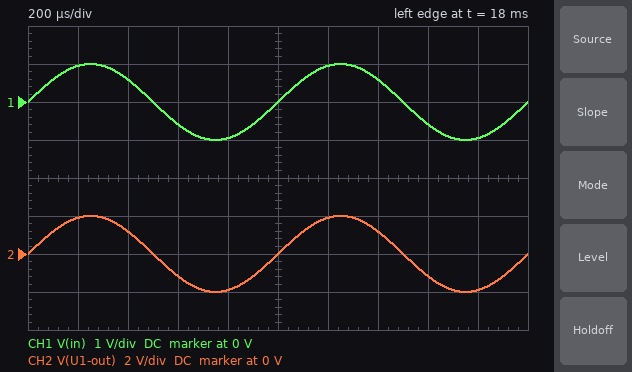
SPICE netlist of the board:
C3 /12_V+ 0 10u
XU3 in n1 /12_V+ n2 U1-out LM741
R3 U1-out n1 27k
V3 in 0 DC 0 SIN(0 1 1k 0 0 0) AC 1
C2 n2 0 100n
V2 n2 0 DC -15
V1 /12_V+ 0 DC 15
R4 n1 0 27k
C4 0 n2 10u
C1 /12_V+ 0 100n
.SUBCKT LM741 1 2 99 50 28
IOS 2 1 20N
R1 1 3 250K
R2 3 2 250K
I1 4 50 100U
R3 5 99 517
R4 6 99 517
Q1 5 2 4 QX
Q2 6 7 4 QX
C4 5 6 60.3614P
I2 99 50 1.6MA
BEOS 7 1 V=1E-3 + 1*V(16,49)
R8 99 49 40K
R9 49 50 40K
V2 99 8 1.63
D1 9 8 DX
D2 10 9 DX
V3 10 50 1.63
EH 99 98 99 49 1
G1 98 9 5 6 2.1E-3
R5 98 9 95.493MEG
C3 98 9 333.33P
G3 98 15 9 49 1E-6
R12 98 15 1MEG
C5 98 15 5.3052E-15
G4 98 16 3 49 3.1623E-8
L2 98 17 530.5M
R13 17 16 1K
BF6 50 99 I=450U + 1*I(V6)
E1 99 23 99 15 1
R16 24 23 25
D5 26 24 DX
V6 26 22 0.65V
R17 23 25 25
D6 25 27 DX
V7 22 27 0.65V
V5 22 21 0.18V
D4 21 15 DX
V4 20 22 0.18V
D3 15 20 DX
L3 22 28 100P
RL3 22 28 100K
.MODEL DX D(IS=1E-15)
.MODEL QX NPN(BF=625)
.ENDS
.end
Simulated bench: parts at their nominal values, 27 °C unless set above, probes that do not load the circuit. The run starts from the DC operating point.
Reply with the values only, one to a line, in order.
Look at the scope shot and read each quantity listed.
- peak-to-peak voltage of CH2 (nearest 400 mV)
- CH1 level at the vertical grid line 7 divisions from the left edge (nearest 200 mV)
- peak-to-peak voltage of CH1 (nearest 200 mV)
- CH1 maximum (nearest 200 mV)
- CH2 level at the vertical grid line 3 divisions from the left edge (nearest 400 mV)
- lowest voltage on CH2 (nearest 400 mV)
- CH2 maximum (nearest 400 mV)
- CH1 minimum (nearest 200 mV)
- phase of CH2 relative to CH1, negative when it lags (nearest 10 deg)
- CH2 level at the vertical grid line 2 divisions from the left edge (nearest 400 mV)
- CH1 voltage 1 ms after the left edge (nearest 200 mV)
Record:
4.0 V
600 mV
2.0 V
1.0 V
-1.2 V
-2.0 V
2.0 V
-1.0 V
0 deg
1.2 V
0 V
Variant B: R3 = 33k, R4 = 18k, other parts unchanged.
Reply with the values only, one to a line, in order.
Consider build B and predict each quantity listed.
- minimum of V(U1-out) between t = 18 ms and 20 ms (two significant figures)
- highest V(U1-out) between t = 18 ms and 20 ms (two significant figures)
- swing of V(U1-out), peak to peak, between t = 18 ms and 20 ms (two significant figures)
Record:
-2.8 V
2.8 V
5.7 V
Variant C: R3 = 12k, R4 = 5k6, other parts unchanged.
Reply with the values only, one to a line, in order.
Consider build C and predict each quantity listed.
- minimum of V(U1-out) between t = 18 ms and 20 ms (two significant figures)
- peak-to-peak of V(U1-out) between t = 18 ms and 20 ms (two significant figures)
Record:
-3.1 V
6.3 V
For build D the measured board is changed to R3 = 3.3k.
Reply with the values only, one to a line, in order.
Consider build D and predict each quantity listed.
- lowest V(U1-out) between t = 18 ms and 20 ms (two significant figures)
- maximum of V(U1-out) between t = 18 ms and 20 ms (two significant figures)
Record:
-1.1 V
1.1 V
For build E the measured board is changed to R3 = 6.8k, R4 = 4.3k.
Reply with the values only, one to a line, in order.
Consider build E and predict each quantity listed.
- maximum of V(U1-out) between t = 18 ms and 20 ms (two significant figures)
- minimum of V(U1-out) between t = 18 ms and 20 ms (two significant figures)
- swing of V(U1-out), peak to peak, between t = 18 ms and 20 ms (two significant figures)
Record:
2.6 V
-2.6 V
5.2 V
